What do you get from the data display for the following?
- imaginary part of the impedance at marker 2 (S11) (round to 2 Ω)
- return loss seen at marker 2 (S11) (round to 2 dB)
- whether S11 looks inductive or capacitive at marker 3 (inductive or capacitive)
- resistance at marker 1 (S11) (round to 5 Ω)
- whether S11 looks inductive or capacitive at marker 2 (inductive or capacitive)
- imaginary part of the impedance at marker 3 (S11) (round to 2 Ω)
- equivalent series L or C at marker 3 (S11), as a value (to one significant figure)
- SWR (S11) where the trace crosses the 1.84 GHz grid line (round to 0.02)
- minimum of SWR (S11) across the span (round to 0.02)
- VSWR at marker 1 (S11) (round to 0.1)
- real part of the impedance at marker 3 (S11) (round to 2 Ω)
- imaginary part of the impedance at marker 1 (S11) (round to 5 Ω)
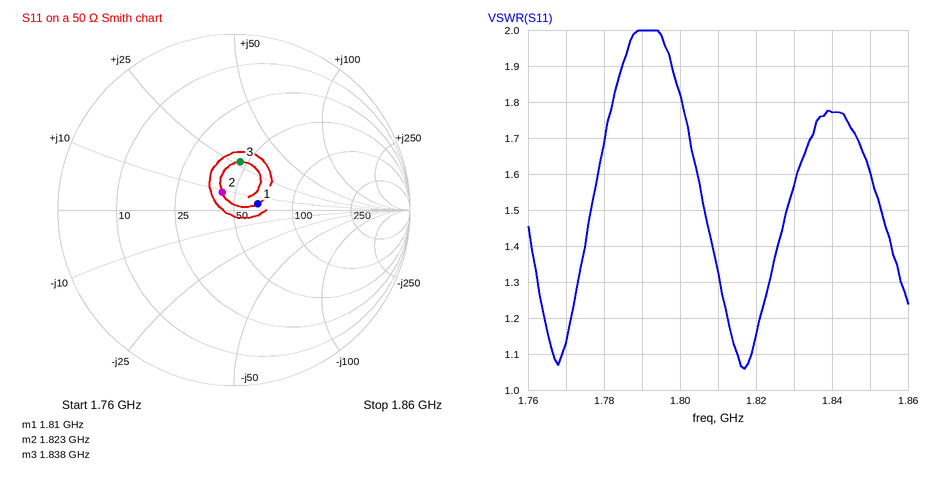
+8 Ω
18 dB
inductive
65 Ω
inductive
+28 Ω
2 nH
1.78
1.06
1.3
46 Ω
+5 Ω
